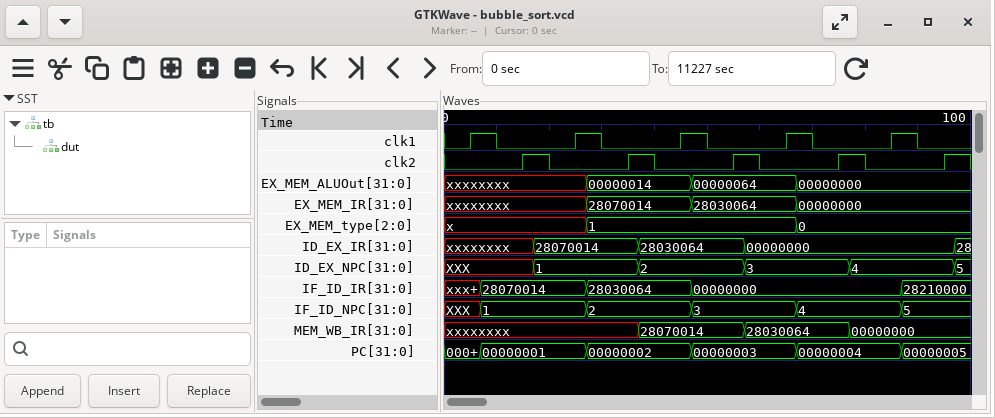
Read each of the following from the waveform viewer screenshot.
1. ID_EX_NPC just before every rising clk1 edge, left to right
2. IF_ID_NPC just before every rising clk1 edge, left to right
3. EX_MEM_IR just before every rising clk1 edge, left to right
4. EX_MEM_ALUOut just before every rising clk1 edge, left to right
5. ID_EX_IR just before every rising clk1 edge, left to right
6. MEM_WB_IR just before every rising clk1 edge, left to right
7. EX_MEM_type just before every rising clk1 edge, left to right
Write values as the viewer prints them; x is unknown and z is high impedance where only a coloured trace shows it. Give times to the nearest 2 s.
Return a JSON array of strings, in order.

["XXX, 1, 2, 3, 4", "XXX, 1, 2, 3, 4", "xxxxxxxx, xxxxxxxx, 28070014, 28030064, 00000000", "xxxxxxxx, xxxxxxxx, 00000014, 00000064, 00000000", "xxxxxxxx, 28070014, 28030064, 00000000, 00000000", "xxxxxxxx, xxxxxxxx, 28070014, 28030064, 00000000", "x, x, 1, 1, 0"]
